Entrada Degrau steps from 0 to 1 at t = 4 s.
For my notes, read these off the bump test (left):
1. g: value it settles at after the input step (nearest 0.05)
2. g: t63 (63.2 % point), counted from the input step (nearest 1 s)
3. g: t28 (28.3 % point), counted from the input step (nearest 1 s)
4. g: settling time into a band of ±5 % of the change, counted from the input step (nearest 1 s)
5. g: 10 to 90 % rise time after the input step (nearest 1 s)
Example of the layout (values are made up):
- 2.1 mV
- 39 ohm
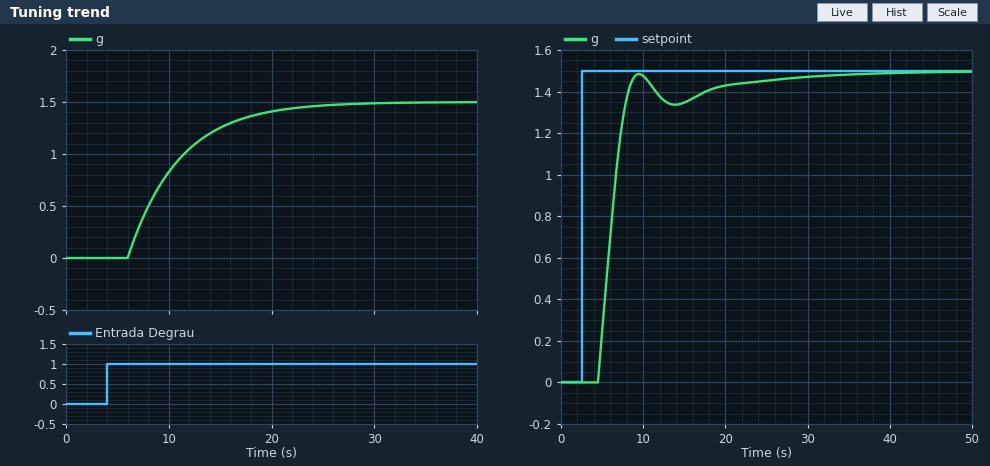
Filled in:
- 1.50
- 7 s
- 4 s
- 17 s
- 11 s
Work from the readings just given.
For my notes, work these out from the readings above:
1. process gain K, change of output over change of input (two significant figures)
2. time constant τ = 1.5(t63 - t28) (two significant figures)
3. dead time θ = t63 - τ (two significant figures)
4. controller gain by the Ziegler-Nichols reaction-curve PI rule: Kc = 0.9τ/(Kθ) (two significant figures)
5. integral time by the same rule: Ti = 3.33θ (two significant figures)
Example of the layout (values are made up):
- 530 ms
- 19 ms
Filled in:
- 1.5
- 4.5 s
- 2.5 s
- 1.1
- 8.3 s
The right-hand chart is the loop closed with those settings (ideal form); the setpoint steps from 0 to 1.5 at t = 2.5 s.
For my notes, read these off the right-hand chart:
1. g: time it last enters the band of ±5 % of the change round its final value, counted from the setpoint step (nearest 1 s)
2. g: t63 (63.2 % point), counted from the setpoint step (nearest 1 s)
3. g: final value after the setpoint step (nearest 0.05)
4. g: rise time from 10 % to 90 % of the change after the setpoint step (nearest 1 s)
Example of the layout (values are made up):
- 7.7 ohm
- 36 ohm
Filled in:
- 17 s
- 4 s
- 1.50
- 3 s
